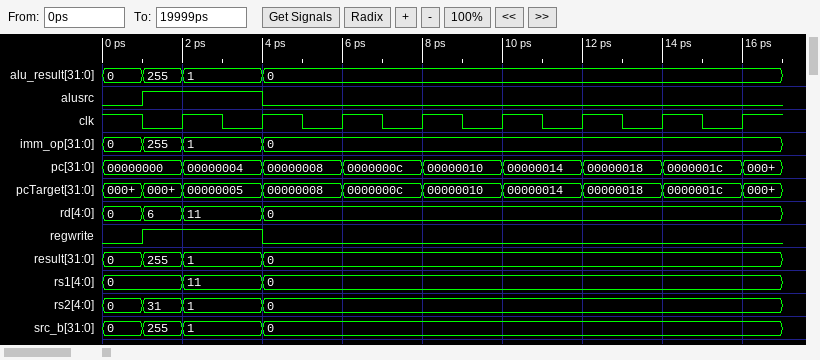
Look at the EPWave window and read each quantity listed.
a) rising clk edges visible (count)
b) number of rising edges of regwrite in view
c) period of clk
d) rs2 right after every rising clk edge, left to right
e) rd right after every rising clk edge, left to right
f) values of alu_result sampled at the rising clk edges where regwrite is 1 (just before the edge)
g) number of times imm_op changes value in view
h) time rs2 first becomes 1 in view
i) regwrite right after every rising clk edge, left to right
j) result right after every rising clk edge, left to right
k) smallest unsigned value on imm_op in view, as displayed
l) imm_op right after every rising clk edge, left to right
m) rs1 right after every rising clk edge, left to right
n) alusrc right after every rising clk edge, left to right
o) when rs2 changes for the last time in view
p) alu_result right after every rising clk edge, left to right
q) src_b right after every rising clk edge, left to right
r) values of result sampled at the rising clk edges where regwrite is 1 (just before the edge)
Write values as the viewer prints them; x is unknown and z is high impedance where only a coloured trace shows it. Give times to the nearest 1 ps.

8
1
2 ps
1, 0, 0, 0, 0, 0, 0, 0
11, 0, 0, 0, 0, 0, 0, 0
255, 1
3
2 ps
1 0 0 0 0 0 0 0
1, 0, 0, 0, 0, 0, 0, 0
0
1, 0, 0, 0, 0, 0, 0, 0
11, 0, 0, 0, 0, 0, 0, 0
1 0 0 0 0 0 0 0
4 ps
1, 0, 0, 0, 0, 0, 0, 0
1, 0, 0, 0, 0, 0, 0, 0
255, 1
